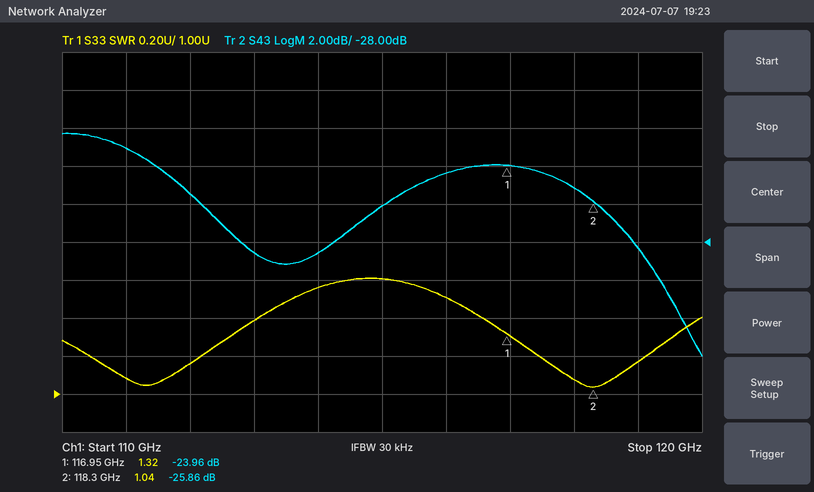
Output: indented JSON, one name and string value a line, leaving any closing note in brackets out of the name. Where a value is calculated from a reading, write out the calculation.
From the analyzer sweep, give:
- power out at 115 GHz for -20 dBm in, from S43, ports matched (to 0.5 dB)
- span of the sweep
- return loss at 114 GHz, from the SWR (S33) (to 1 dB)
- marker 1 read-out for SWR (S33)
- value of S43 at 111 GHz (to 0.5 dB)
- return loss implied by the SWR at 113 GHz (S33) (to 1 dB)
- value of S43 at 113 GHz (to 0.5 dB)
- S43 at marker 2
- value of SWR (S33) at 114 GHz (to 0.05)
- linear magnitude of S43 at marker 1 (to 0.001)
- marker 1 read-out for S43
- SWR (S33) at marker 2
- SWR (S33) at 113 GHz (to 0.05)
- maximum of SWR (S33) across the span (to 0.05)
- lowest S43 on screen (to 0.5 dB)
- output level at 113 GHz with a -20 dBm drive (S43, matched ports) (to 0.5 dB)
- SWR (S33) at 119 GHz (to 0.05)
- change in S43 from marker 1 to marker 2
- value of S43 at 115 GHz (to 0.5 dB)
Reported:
{
  "power out at 115 GHz for -20 dBm in, from S43, ports matched": "-20 dBm + (-26.0 dB) = -46.0 dBm",
  "span of the sweep": "10 GHz",
  "return loss at 114 GHz, from the SWR (S33)": "−20 log10((1.55 − 1)/(1.55 + 1)) ≈ 13 dB",
  "marker 1 read-out for SWR": "1.32",
  "value of S43 at 111 GHz": "-23.0 dB",
  "return loss implied by the SWR at 113 GHz (S33)": "−20 log10((1.4 − 1)/(1.4 + 1)) ≈ 16 dB",
  "value of S43 at 113 GHz": "-28.5 dB",
  "S43 at marker 2": "-25.86 dB",
  "value of SWR (S33) at 114 GHz": "1.55",
  "linear magnitude of S43 at marker 1": "10^(-23.96/20) ≈ 0.063",
  "marker 1 read-out for S43": "-23.96 dB",
  "SWR (S33) at marker 2": "1.04",
  "SWR (S33) at 113 GHz": "1.40",
  "maximum of SWR (S33) across the span": "1.60",
  "lowest S43 on screen": "-34.0 dB",
  "output level at 113 GHz with a -20 dBm drive (S43, matched ports)": "-20 dBm + (-28.5 dB) = -48.5 dBm",
  "SWR (S33) at 119 GHz": "1.15",
  "change in S43 from marker 1 to marker 2": "-25.86 − (-23.96) = -1.90 dB",
  "value of S43 at 115 GHz": "-26.0 dB"
}
